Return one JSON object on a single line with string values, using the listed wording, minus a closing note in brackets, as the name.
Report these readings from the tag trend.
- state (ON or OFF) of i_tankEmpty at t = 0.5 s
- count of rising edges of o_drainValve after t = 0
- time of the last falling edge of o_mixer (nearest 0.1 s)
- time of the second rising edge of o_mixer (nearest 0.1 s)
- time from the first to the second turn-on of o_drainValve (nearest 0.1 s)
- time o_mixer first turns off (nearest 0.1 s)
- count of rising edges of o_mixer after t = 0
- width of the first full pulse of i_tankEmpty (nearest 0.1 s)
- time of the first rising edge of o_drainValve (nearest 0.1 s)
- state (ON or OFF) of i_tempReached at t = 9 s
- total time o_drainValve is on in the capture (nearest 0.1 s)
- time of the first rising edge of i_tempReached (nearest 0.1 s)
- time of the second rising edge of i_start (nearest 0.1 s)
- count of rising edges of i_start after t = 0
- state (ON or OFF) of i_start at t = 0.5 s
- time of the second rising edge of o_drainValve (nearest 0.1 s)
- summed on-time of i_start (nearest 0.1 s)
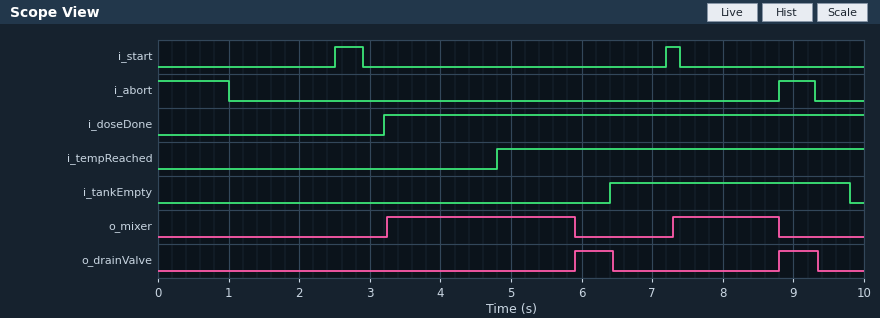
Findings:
{"state (ON or OFF) of i_tankEmpty at t = 0.5 s": "OFF", "count of rising edges of o_drainValve after t = 0": "2", "time of the last falling edge of o_mixer": "8.8 s", "time of the second rising edge of o_mixer": "7.3 s", "time from the first to the second turn-on of o_drainValve": "2.9 s", "time o_mixer first turns off": "5.9 s", "count of rising edges of o_mixer after t = 0": "2", "width of the first full pulse of i_tankEmpty": "3.4 s", "time of the first rising edge of o_drainValve": "5.9 s", "state (ON or OFF) of i_tempReached at t = 9 s": "ON", "total time o_drainValve is on in the capture": "1.1 s", "time of the first rising edge of i_tempReached": "4.8 s", "time of the second rising edge of i_start": "7.2 s", "count of rising edges of i_start after t = 0": "2", "state (ON or OFF) of i_start at t = 0.5 s": "OFF", "time of the second rising edge of o_drainValve": "8.8 s", "summed on-time of i_start": "0.6 s"}
